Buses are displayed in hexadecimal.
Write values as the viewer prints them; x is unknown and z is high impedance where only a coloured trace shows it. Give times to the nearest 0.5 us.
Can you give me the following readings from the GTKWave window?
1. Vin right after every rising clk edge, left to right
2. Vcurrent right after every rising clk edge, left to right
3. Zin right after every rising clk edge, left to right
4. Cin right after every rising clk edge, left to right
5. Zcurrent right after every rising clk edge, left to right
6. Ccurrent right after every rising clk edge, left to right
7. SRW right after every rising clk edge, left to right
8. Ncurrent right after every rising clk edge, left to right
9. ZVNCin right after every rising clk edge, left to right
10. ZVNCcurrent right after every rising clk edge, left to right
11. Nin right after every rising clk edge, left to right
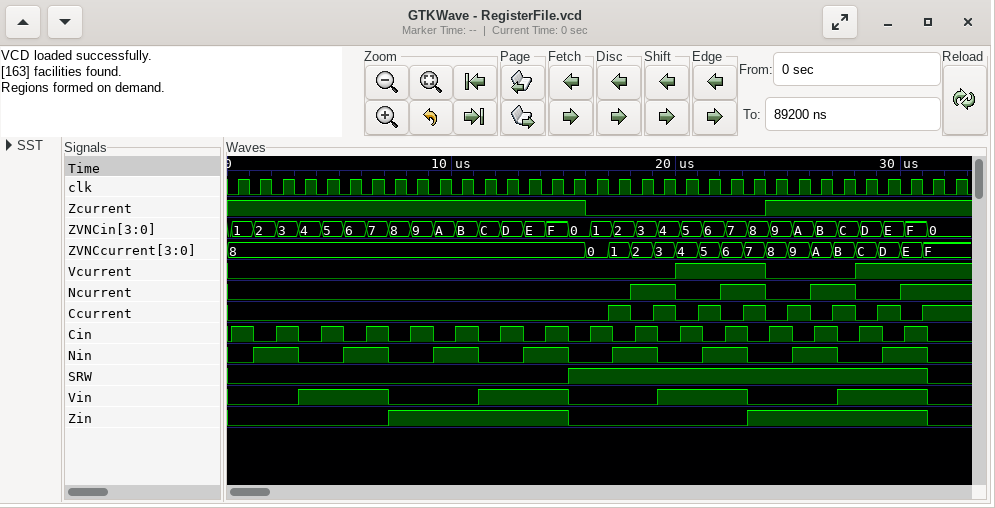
0 0 0 1 1 1 1 0 0 0 0 1 1 1 1 0 0 0 0 1 1 1 1 0 0 0 0 1 1 1 1 0 0
0 0 0 0 0 0 0 0 0 0 0 0 0 0 0 0 0 0 0 0 1 1 1 1 0 0 0 0 1 1 1 1 1
0 0 0 0 0 0 0 1 1 1 1 1 1 1 1 0 0 0 0 0 0 0 0 1 1 1 1 1 1 1 1 0 0
1 0 1 0 1 0 1 0 1 0 1 0 1 0 1 0 1 0 1 0 1 0 1 0 1 0 1 0 1 0 1 0 0
1 1 1 1 1 1 1 1 1 1 1 1 1 1 1 1 0 0 0 0 0 0 0 0 1 1 1 1 1 1 1 1 1
0 0 0 0 0 0 0 0 0 0 0 0 0 0 0 0 0 1 0 1 0 1 0 1 0 1 0 1 0 1 0 1 1
0 0 0 0 0 0 0 0 0 0 0 0 0 0 0 1 1 1 1 1 1 1 1 1 1 1 1 1 1 1 1 0 0
0 0 0 0 0 0 0 0 0 0 0 0 0 0 0 0 0 0 1 1 0 0 1 1 0 0 1 1 0 0 1 1 1
1, 2, 3, 4, 5, 6, 7, 8, 9, A, B, C, D, E, F, 0, 1, 2, 3, 4, 5, 6, 7, 8, 9, A, B, C, D, E, F, 0, 0
8, 8, 8, 8, 8, 8, 8, 8, 8, 8, 8, 8, 8, 8, 8, 8, 0, 1, 2, 3, 4, 5, 6, 7, 8, 9, A, B, C, D, E, F, F
0 1 1 0 0 1 1 0 0 1 1 0 0 1 1 0 0 1 1 0 0 1 1 0 0 1 1 0 0 1 1 0 0
